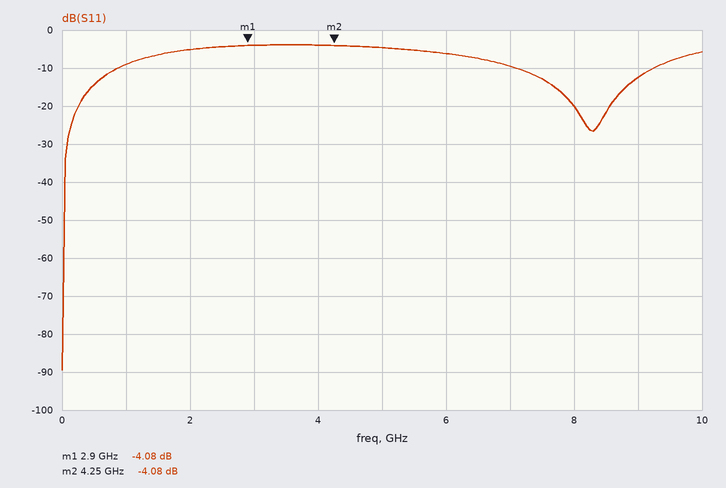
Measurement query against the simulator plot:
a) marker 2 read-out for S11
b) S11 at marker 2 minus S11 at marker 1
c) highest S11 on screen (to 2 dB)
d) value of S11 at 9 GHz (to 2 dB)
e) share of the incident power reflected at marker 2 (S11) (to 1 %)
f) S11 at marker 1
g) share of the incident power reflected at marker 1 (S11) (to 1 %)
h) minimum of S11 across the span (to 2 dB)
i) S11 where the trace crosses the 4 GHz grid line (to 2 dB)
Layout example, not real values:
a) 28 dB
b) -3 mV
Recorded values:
a) -4.08 dB
b) 0.00 dB
c) -4 dB
d) -12 dB
e) 39 %
f) -4.08 dB
g) 39 %
h) -90 dB
i) -4 dB
